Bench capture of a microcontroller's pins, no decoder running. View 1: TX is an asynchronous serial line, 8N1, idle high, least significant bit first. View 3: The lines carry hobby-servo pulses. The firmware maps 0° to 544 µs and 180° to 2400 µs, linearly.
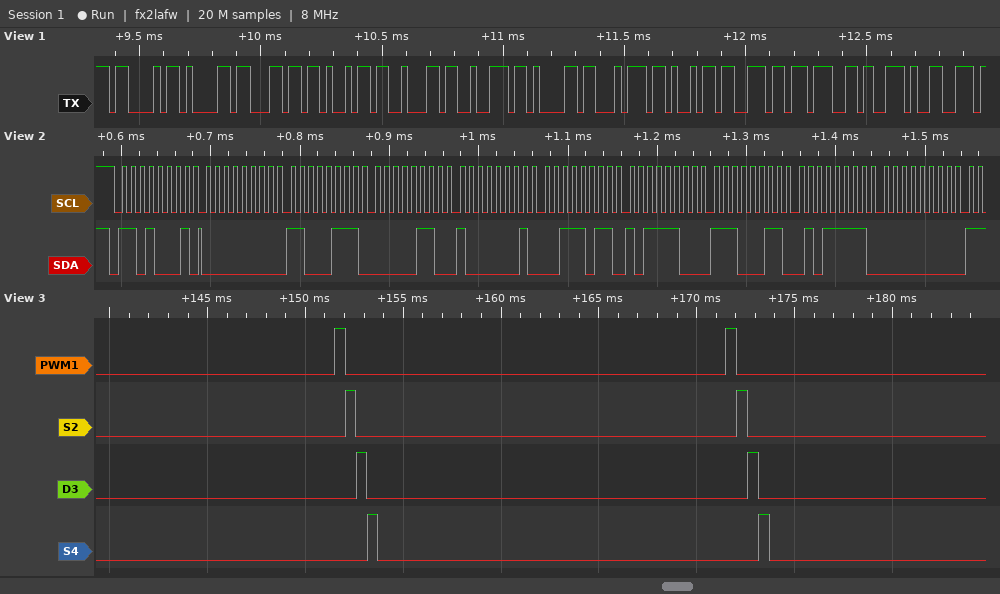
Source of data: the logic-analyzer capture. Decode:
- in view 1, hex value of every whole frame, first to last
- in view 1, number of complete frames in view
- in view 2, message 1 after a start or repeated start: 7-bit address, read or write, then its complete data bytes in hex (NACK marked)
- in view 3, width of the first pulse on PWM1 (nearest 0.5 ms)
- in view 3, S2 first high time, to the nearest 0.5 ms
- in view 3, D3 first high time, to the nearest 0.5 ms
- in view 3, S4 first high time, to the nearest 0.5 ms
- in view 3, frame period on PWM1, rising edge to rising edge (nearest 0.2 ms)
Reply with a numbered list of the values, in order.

1. 43 61 6C 69 62 72 61 74 69 6E 67 2E
2. 12
3. 0x68 read: 00 C7 06 81 3B BC E3 5F 00
4. 0.5 ms
5. 0.5 ms
6. 0.5 ms
7. 0.5 ms
8. 20.0 ms
